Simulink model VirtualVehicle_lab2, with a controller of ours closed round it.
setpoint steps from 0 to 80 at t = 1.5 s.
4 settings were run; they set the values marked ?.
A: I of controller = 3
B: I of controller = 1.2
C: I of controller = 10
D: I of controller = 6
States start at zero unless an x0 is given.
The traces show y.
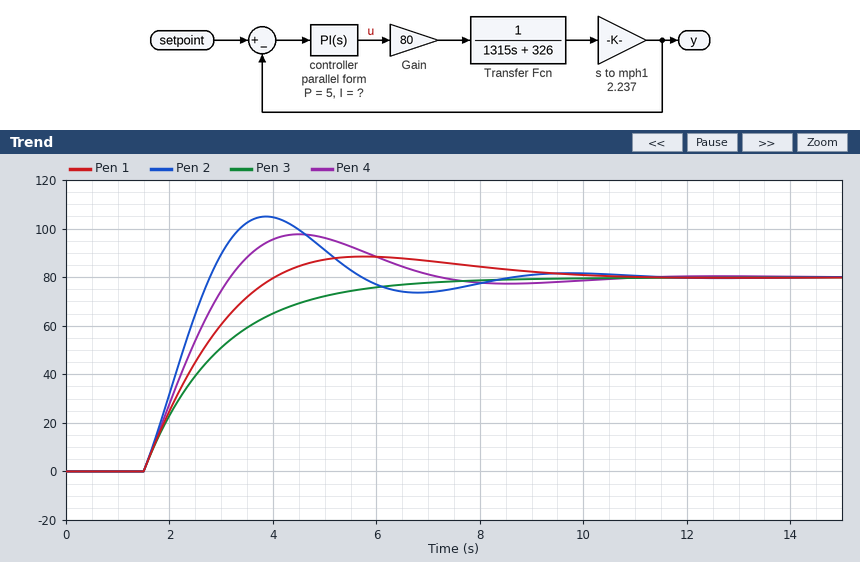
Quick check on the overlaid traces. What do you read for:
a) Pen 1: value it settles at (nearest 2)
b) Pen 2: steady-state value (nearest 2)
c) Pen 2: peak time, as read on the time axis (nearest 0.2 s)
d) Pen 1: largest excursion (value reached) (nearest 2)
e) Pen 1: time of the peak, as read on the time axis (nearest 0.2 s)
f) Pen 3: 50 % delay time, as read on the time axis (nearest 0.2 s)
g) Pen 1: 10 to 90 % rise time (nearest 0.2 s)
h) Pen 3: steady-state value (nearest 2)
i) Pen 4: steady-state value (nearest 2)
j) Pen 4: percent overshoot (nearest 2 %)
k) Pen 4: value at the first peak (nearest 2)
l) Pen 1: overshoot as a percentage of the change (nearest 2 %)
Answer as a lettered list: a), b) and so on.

a) 80
b) 80
c) 3.8 s
d) 88
e) 5.8 s
f) 2.6 s
g) 1.8 s
h) 80
i) 80
j) 22 %
k) 98
l) 10 %
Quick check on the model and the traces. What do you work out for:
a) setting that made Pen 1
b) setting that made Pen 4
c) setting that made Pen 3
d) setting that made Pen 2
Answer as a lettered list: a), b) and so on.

a) A
b) D
c) B
d) C
